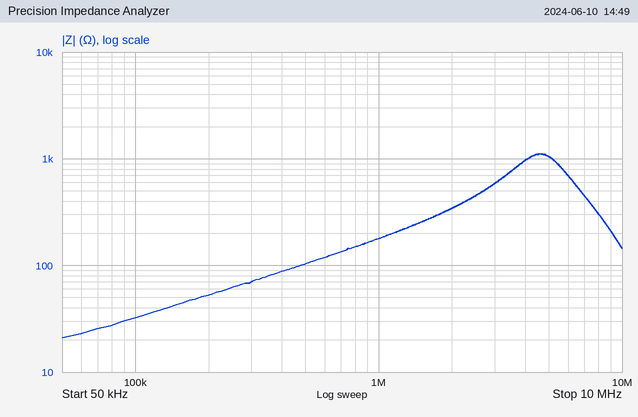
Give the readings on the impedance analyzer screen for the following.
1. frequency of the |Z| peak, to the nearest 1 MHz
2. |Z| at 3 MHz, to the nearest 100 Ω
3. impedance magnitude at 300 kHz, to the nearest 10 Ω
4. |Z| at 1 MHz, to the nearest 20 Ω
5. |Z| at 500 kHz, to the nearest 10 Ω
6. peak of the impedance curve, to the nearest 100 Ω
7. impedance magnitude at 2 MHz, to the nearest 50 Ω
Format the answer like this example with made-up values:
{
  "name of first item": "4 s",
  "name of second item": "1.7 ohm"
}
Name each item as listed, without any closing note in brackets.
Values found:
{
  "frequency of the |Z| peak, to the nearest 1 MHz": "5 MHz",
  "|Z| at 3 MHz, to the nearest 100 Ω": "600 Ω",
  "impedance magnitude at 300 kHz, to the nearest 10 Ω": "70 Ω",
  "|Z| at 1 MHz, to the nearest 20 Ω": "180 Ω",
  "|Z| at 500 kHz, to the nearest 10 Ω": "100 Ω",
  "peak of the impedance curve, to the nearest 100 Ω": "1.1 kΩ",
  "impedance magnitude at 2 MHz, to the nearest 50 Ω": "350 Ω"
}
